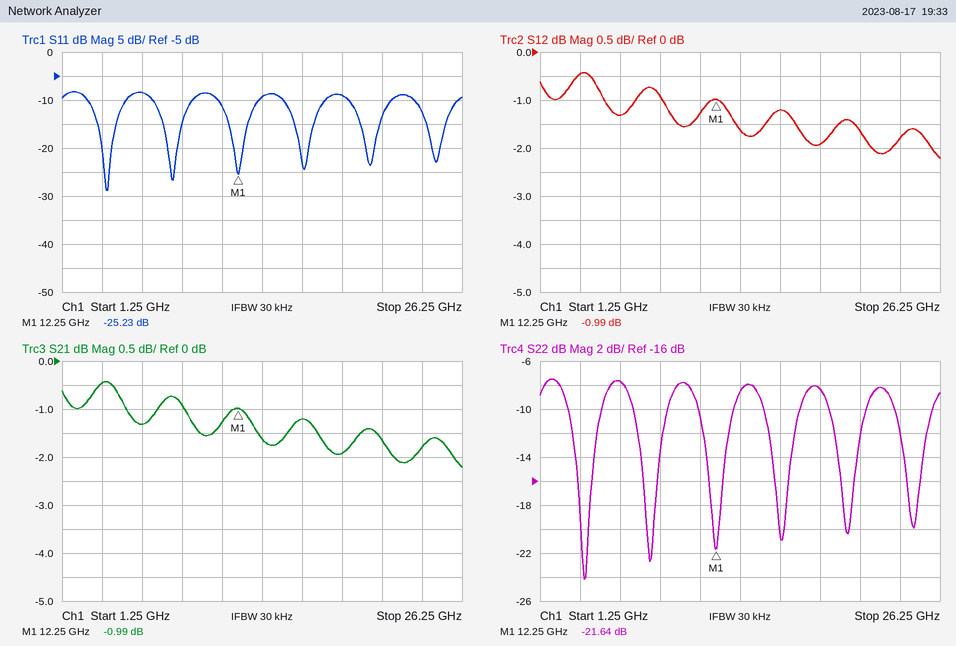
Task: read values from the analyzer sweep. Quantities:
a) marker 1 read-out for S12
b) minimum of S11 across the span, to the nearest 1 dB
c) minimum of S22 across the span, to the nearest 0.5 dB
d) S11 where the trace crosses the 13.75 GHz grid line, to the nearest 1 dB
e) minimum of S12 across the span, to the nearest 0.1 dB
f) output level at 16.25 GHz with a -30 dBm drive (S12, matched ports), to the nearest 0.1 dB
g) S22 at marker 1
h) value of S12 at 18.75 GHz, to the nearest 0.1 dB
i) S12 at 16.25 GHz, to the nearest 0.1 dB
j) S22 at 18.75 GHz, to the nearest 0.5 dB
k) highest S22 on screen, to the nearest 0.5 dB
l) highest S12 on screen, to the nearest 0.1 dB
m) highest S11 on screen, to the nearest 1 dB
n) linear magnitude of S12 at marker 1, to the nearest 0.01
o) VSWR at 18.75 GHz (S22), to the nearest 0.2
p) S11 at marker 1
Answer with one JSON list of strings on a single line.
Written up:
["-0.99 dB", "-29 dB", "-24.0 dB", "-9 dB", "-2.2 dB", "-31.2 dBm", "-21.64 dB", "-1.9 dB", "-1.2 dB", "-8.5 dB", "-7.5 dB", "-0.4 dB", "-8 dB", "0.89", "2.2", "-25.23 dB"]
